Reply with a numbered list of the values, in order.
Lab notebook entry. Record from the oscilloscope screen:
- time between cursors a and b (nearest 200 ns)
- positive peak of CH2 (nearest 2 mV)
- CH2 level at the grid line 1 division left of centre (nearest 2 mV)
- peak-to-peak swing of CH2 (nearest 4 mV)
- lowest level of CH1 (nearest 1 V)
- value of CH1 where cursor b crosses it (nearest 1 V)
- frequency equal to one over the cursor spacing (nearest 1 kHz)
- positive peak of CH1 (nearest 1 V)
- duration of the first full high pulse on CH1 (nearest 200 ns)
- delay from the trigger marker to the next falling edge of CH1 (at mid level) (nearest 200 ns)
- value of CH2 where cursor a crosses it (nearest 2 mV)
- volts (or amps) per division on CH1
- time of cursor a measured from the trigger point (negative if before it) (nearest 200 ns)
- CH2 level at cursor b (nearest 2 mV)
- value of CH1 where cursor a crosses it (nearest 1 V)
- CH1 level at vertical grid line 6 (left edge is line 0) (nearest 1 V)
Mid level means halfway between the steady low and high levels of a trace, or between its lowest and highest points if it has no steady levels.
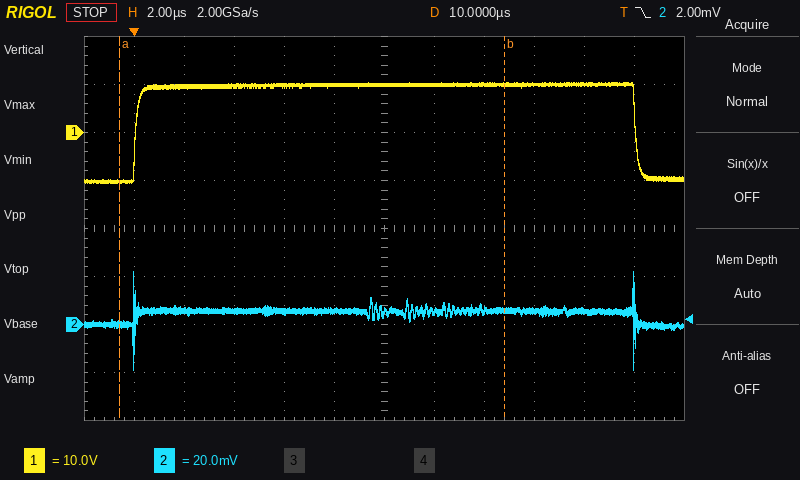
1. 15.4 µs
2. 22 mV
3. 6 mV
4. 40 mV
5. -10 V
6. 10 V
7. 65 kHz
8. 10 V
9. 20.0 µs
10. 20.0 µs
11. 0 mV
12. 10 V
13. -600 ns
14. 6 mV
15. -10 V
16. 10 V
